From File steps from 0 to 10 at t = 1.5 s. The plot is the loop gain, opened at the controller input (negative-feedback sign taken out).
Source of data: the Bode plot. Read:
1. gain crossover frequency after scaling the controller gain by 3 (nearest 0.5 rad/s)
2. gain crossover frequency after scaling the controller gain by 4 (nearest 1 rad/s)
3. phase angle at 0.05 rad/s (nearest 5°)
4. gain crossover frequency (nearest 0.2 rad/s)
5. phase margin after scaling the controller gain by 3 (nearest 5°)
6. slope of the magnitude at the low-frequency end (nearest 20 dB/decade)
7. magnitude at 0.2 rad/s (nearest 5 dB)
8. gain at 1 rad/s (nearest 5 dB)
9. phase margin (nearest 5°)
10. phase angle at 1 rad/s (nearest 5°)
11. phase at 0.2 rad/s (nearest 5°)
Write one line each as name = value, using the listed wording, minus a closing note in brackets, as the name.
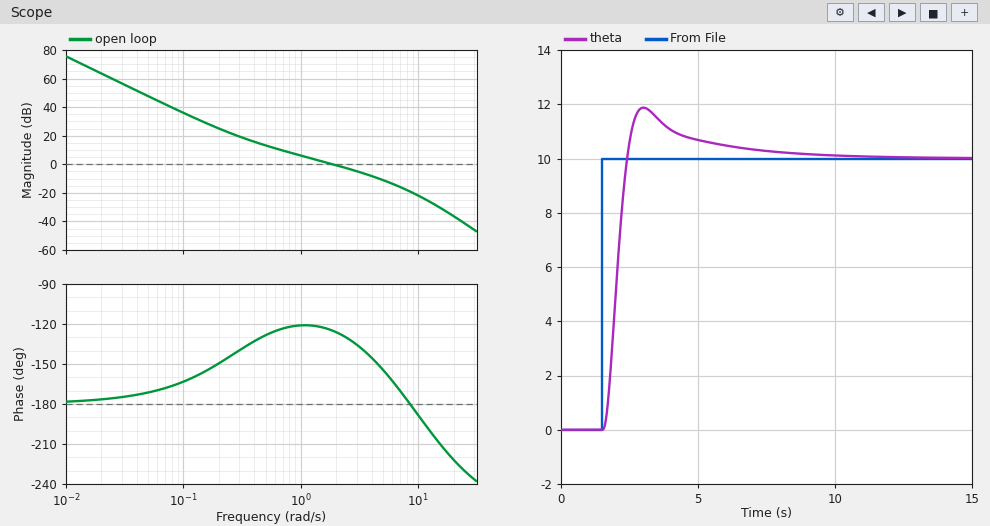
gain crossover frequency after scaling the controller gain by 3 = 4.5 rad/s
gain crossover frequency after scaling the controller gain by 4 = 5 rad/s
phase angle at 0.05 rad/s = -170°
gain crossover frequency = 1.8 rad/s
phase margin after scaling the controller gain by 3 = 30°
slope of the magnitude at the low-frequency end = -40 dB/decade
magnitude at 0.2 rad/s = 25 dB
gain at 1 rad/s = 5 dB
phase margin = 55°
phase angle at 1 rad/s = -120°
phase at 0.2 rad/s = -150°
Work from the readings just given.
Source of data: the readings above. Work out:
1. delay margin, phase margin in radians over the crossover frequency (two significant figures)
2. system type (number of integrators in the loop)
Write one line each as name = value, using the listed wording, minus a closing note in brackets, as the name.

delay margin, phase margin in radians over the crossover frequency = 0.53 s
system type = 2
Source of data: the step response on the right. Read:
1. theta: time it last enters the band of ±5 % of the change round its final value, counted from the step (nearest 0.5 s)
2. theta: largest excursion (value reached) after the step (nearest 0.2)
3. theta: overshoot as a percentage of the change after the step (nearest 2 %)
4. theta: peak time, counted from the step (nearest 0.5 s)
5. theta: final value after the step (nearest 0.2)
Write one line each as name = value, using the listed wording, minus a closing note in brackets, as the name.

theta: time it last enters the band of ±5 % of the change round its final value, counted from the step = 4.5 s
theta: largest excursion (value reached) after the step = 11.8
theta: overshoot as a percentage of the change after the step = 18 %
theta: peak time, counted from the step = 1.5 s
theta: final value after the step = 10.0
